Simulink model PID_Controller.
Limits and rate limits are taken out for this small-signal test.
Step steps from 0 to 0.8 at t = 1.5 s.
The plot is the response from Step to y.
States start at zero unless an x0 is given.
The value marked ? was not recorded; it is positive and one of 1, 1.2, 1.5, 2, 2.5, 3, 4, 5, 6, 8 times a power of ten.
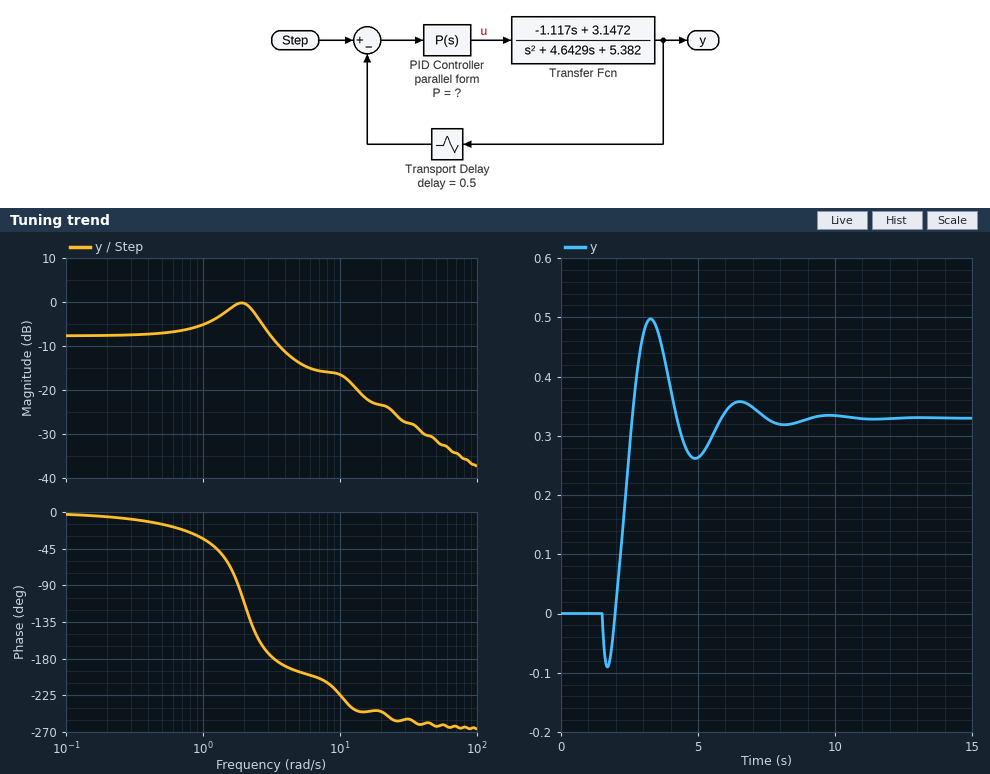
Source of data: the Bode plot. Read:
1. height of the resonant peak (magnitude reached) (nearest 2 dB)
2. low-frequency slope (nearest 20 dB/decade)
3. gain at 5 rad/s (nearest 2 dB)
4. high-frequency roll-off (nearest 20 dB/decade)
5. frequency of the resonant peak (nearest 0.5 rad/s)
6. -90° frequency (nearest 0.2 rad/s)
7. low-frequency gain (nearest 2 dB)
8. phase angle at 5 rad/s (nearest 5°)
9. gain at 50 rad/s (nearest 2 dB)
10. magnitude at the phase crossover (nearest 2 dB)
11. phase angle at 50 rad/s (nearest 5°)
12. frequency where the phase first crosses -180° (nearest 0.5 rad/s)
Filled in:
0 dB
0 dB/decade
-14 dB
-20 dB/decade
2.0 rad/s
1.8 rad/s
-8 dB
-195°
-32 dB
-8 dB
-265°
3.5 rad/s
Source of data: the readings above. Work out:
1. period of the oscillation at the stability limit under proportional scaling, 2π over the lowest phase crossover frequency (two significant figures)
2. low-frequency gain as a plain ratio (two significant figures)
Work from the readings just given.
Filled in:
1.8 s
0.40
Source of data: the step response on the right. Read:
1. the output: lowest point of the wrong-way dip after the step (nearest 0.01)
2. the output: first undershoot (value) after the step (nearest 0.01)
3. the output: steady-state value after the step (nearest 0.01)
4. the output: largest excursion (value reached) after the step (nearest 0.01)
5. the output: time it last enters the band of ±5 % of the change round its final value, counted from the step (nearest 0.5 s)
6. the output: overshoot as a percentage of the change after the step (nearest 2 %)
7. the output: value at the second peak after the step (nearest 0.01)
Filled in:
-0.09
0.26
0.33
0.50
5.5 s
50 %
0.36
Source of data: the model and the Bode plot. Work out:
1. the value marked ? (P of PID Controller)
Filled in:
1.2
